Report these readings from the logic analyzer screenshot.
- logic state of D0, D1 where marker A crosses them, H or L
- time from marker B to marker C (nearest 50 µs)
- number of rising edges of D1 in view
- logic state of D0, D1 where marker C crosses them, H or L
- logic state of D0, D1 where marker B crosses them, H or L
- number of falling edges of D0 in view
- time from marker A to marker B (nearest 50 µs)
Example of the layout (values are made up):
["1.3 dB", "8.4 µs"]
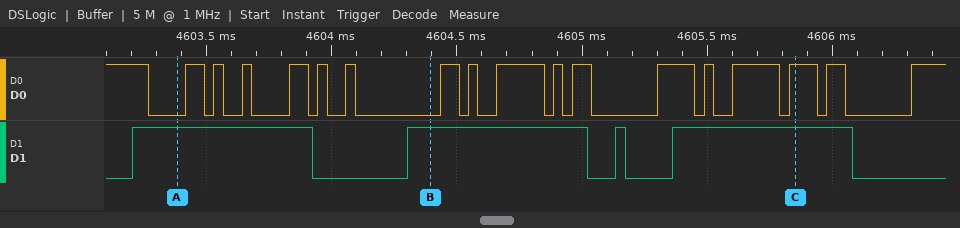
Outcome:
["D0=L, D1=H", "1450 µs", "4", "D0=H, D1=H", "D0=L, D1=H", "17", "1000 µs"]
